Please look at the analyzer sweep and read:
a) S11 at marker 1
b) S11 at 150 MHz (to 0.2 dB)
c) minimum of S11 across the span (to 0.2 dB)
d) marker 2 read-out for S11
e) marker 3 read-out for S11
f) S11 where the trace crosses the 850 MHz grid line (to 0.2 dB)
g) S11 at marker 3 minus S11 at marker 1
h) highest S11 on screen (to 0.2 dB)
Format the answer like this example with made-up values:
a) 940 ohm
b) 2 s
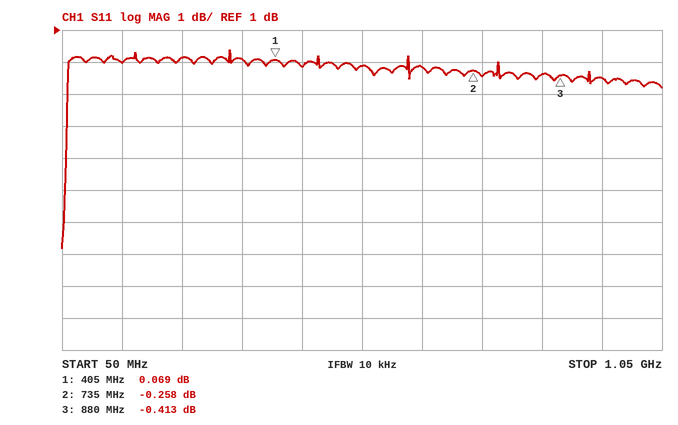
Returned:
a) 0.069 dB
b) 0.0 dB
c) -5.8 dB
d) -0.258 dB
e) -0.413 dB
f) -0.4 dB
g) -0.482 dB
h) 0.4 dB
